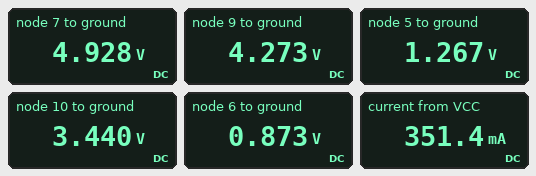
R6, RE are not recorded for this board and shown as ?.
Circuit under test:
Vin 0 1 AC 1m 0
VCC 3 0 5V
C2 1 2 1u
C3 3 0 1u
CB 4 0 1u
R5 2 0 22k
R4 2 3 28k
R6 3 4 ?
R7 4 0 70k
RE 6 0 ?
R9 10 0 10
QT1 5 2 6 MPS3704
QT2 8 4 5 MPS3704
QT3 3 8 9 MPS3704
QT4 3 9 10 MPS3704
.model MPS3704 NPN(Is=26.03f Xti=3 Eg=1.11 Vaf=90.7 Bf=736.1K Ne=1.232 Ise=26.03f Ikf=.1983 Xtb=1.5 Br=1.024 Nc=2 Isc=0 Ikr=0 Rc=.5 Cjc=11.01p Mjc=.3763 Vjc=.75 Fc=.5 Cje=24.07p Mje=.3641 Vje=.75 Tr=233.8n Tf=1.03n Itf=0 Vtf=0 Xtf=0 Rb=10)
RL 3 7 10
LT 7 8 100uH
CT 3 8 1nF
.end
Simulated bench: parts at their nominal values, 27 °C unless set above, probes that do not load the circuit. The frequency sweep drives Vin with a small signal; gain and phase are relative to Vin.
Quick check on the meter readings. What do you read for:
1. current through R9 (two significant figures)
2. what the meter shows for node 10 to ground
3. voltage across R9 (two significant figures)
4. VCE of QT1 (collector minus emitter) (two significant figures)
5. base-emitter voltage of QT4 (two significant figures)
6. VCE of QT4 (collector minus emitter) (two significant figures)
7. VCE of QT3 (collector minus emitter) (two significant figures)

340 mA
3.440 V
3.4 V
390 mV
830 mV
1.6 V
730 mV
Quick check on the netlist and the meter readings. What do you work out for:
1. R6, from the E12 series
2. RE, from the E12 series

39 kΩ
120 Ω
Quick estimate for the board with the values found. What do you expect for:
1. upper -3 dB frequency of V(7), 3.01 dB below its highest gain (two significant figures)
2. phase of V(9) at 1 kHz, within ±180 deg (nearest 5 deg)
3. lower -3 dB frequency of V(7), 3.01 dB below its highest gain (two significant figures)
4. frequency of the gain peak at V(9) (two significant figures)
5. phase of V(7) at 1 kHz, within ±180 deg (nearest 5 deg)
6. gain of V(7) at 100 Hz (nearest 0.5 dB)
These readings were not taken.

510 kHz
5 deg
490 kHz
500 kHz
0 deg
-22.0 dB
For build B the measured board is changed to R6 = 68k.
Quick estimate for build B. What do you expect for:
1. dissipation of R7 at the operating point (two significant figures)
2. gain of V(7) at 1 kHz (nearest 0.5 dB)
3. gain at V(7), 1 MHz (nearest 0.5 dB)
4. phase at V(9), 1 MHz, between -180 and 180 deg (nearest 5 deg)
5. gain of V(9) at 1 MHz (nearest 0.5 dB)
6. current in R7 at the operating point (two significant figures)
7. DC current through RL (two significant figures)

26 µW
-25.0 dB
-33.5 dB
-115 deg
2.5 dB
19 µA
4.6 mA
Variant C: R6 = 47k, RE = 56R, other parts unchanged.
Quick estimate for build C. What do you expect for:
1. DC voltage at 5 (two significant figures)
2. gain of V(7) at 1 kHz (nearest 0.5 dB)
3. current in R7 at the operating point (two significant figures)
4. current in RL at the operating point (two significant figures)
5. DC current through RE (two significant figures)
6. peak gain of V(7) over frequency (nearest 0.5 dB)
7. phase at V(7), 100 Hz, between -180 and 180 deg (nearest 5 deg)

650 mV
-16.0 dB
19 µA
8.7 mA
8.8 mA
13.5 dB
65 deg
